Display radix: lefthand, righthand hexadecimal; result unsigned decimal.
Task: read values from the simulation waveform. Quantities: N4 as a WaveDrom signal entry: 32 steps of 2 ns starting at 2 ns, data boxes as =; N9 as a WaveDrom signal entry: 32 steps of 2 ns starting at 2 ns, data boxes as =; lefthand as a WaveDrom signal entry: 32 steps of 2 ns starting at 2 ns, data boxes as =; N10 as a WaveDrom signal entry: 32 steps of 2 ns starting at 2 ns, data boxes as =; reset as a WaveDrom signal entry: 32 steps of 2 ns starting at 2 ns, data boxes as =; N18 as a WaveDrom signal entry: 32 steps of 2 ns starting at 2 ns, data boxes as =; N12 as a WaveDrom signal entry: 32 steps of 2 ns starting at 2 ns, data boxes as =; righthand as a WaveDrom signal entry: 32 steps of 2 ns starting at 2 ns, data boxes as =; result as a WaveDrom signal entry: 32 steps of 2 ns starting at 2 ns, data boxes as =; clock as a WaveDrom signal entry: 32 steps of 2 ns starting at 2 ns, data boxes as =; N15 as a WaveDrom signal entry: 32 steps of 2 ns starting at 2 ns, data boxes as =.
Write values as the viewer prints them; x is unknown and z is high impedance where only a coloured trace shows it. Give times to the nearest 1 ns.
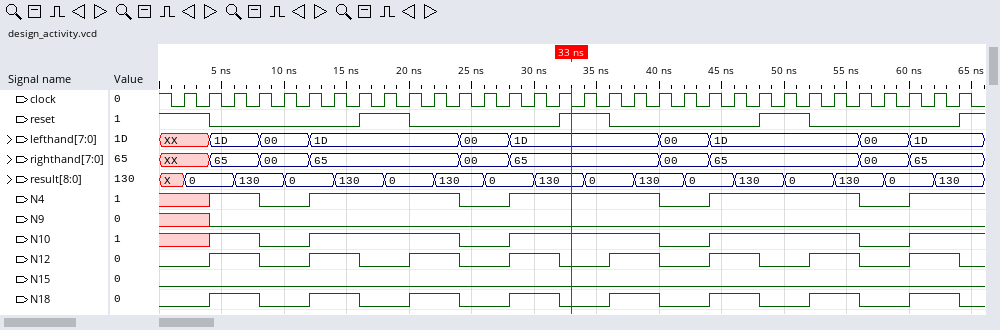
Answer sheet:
{name: 'N4', wave: 'x1.0.1.....0.1.....0.1.....0.1..'}
{name: 'N9', wave: 'x0..............................'}
{name: 'lefthand', wave: 'x=.=.=.....=.=.....=.=.....=.=..', data: '1D 00 1D 00 1D 00 1D 00 1D'}
{name: 'N10', wave: 'x1.0.1.....0.1.....0.1.....0.1..'}
{name: 'reset', wave: '10.....1.0.....1.0.....1.0.....1'}
{name: 'N18', wave: '01.0.1.0.1.0.1.0.1.0.1.0.1.0.1.0'}
{name: 'N12', wave: '01.0.1.0.1.0.1.0.1.0.1.0.1.0.1.0'}
{name: 'righthand', wave: 'x=.=.=.....=.=.....=.=.....=.=..', data: '65 00 65 00 65 00 65 00 65'}
{name: 'result', wave: '=.=.=.=.=.=.=.=.=.=.=.=.=.=.=.=.', data: '0 130 0 130 0 130 0 130 0 130 0 130 0 130 0 130'}
{name: 'clock', wave: 'p...............................'}
{name: 'N15', wave: '0...............................'}
